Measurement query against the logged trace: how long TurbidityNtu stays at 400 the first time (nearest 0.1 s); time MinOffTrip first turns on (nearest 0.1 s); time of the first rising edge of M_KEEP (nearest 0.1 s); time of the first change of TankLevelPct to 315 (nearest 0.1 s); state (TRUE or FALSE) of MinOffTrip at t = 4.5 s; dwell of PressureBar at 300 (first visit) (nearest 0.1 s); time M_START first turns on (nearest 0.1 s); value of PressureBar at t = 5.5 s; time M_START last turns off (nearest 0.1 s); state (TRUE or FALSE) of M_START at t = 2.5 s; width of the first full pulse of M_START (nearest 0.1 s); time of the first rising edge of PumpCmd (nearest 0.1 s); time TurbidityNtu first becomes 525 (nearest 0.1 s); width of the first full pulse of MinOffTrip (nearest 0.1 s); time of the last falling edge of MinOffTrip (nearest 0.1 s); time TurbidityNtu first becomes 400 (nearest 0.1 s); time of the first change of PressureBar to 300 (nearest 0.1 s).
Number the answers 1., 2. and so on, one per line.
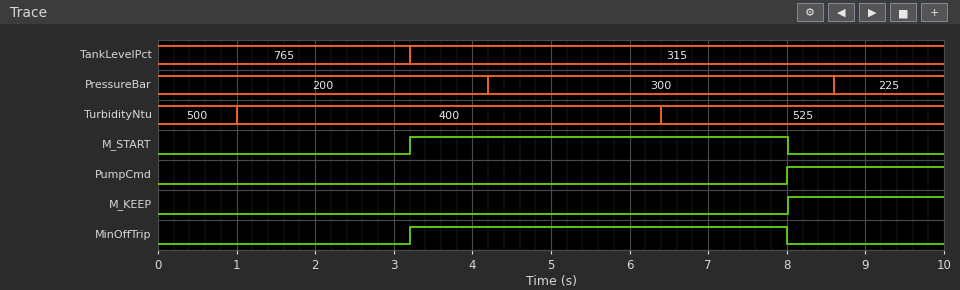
1. 5.4 s
2. 3.2 s
3. 8.0 s
4. 3.2 s
5. TRUE
6. 4.4 s
7. 3.2 s
8. 300
9. 8.0 s
10. FALSE
11. 4.8 s
12. 8.0 s
13. 6.4 s
14. 4.8 s
15. 8.0 s
16. 1.0 s
17. 4.2 s
